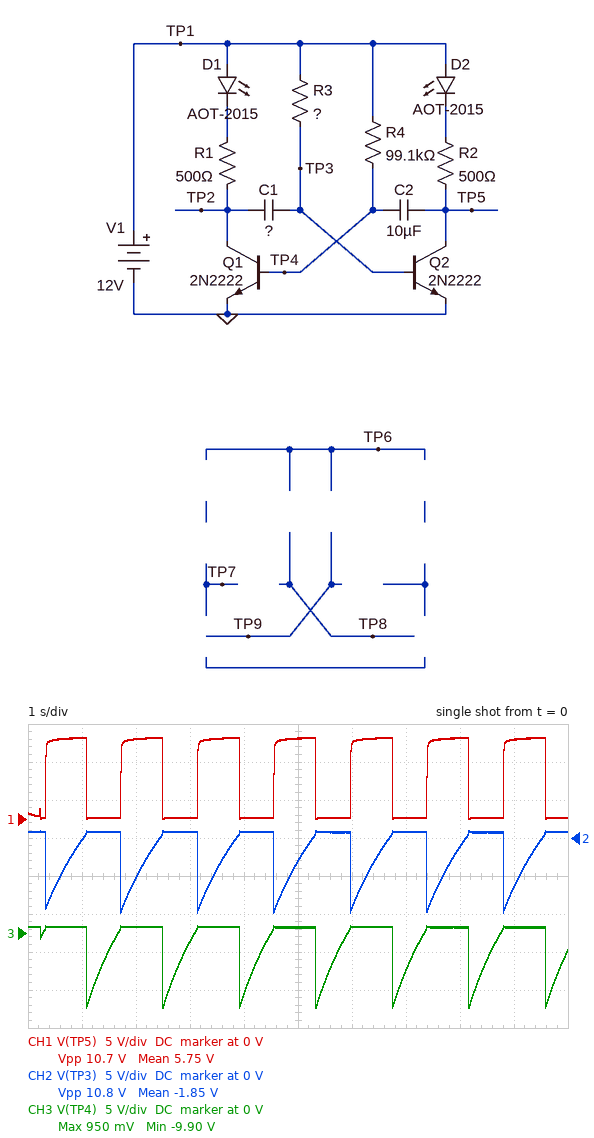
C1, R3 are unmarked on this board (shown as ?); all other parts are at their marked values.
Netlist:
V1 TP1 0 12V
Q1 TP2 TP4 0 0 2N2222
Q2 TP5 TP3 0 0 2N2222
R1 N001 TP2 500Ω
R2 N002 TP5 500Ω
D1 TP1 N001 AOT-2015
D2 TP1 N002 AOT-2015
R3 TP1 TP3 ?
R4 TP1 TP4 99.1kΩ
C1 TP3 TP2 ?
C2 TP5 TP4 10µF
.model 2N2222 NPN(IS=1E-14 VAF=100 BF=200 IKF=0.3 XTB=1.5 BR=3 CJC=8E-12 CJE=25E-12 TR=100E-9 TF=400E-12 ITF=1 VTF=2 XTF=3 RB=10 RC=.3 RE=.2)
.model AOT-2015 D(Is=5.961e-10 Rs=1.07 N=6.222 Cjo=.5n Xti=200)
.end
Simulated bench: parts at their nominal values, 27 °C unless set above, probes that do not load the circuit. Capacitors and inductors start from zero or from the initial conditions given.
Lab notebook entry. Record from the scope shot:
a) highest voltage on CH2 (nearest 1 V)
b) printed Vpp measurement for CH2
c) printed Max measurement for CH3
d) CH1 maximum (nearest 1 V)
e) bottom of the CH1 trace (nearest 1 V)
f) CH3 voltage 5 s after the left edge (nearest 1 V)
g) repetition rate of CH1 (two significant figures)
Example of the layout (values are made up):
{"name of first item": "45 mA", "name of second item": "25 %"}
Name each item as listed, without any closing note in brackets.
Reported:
{"highest voltage on CH2": "1 V", "printed Vpp measurement for CH2": "10.8 V", "printed Max measurement for CH3": "950 mV", "CH1 maximum": "11 V", "bottom of the CH1 trace": "0 V", "CH3 voltage 5 s after the left edge": "1 V", "repetition rate of CH1": "710 mHz"}
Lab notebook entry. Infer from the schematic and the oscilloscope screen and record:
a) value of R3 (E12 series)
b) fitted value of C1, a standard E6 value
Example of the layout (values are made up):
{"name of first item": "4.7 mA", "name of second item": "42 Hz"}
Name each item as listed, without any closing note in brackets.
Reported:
{"value of R3": "82 kΩ", "fitted value of C1, a standard E6 value": "15 µF"}
